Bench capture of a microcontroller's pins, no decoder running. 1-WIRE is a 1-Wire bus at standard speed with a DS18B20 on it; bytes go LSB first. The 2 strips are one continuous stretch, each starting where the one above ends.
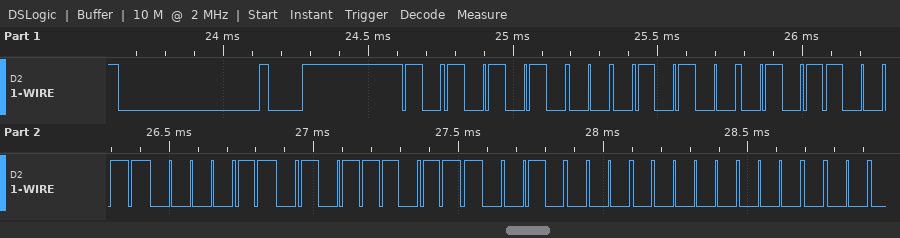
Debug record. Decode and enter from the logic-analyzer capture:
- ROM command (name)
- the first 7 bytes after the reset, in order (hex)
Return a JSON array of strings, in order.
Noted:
["Match ROM", "55 28 9A 61 DD 09 00"]
